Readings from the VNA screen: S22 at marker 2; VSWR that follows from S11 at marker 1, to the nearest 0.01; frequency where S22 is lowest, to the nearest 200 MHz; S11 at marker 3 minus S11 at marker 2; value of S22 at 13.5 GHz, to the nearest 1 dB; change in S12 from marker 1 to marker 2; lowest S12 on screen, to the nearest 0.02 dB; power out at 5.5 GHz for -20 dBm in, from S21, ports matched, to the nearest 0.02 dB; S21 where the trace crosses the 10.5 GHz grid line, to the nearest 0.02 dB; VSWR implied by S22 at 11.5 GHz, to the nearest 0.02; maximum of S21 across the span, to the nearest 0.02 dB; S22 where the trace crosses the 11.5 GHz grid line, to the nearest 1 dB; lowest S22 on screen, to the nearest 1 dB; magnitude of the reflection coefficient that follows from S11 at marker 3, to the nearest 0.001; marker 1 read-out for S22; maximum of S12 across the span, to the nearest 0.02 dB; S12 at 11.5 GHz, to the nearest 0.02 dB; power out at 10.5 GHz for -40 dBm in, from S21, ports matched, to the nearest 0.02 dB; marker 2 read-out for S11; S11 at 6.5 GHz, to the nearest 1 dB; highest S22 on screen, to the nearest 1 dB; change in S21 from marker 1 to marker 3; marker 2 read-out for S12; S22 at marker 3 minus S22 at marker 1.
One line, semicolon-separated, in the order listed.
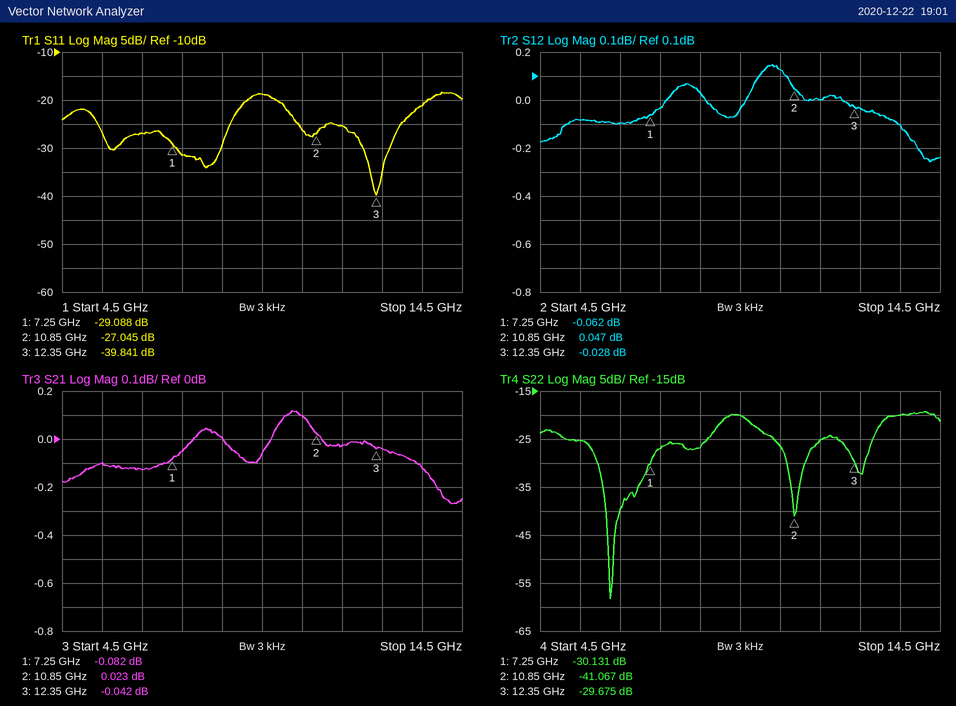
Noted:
-41.067 dB; 1.07; 6.2 GHz; -12.796 dB; -20 dB; 0.109 dB; -0.26 dB; -20.10 dBm; 0.10 dB; 1.12; 0.12 dB; -25 dB; -58 dB; 0.010; -30.131 dB; 0.14 dB; 0.00 dB; -39.90 dBm; -27.045 dB; -27 dB; -19 dB; 0.040 dB; 0.047 dB; 0.456 dB
